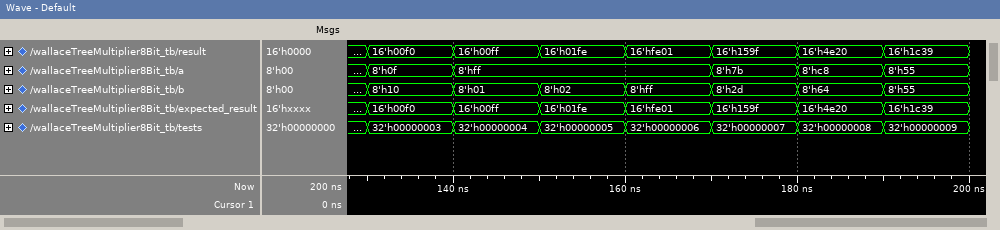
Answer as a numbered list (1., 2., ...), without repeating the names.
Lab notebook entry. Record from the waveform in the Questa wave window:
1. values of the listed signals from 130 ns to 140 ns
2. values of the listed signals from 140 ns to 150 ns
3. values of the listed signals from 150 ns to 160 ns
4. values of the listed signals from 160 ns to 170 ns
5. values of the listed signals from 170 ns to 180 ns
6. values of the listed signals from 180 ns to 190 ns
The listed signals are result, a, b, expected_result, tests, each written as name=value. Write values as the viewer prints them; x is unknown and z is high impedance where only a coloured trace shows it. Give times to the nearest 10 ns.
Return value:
1. result=16'h00f0, a=8'h0f, b=8'h10, expected_result=16'h00f0, tests=32'h00000003
2. result=16'h00ff, a=8'hff, b=8'h01, expected_result=16'h00ff, tests=32'h00000004
3. result=16'h01fe, a=8'hff, b=8'h02, expected_result=16'h01fe, tests=32'h00000005
4. result=16'hfe01, a=8'hff, b=8'hff, expected_result=16'hfe01, tests=32'h00000006
5. result=16'h159f, a=8'h7b, b=8'h2d, expected_result=16'h159f, tests=32'h00000007
6. result=16'h4e20, a=8'hc8, b=8'h64, expected_result=16'h4e20, tests=32'h00000008
